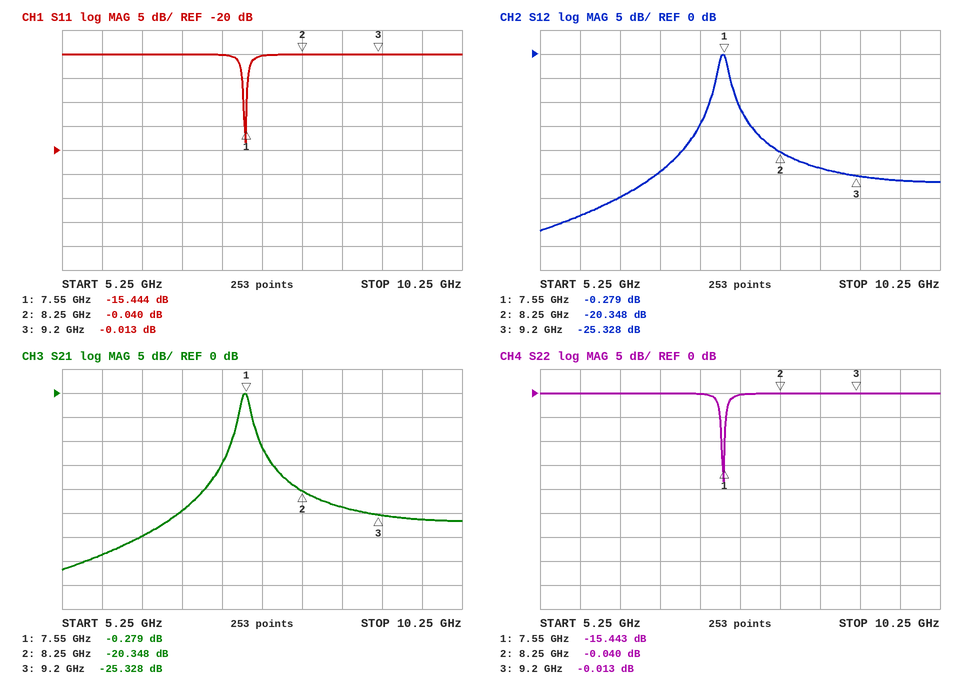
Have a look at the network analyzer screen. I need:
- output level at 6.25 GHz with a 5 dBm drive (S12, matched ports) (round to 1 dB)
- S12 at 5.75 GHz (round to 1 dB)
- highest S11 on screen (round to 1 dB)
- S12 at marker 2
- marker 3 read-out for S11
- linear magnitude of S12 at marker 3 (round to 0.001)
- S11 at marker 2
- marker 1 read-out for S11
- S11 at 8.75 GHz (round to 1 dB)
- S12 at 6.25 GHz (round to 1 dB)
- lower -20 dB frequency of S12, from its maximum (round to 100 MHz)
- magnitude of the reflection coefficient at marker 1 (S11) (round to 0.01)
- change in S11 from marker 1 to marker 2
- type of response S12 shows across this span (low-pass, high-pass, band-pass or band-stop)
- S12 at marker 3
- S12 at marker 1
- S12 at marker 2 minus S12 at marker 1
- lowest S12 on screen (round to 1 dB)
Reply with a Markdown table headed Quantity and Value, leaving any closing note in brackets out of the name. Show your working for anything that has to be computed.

| Quantity | Value |
|---|---|
| output level at 6.25 GHz with a 5 dBm drive (S12, matched ports) | 5 dBm + (-30 dB) = -25 dBm |
| S12 at 5.75 GHz | -34 dB |
| highest S11 on screen | 0 dB |
| S12 at marker 2 | -20.348 dB |
| marker 3 read-out for S11 | -0.013 dB |
| linear magnitude of S12 at marker 3 | 10^(-25.328/20) ≈ 0.054 |
| S11 at marker 2 | -0.040 dB |
| marker 1 read-out for S11 | -15.444 dB |
| S11 at 8.75 GHz | 0 dB |
| S12 at 6.25 GHz | -30 dB |
| lower -20 dB frequency of S12, from its maximum | 7.0 GHz |
| magnitude of the reflection coefficient at marker 1 (S11) | 10^(-15.444/20) ≈ 0.17 |
| change in S11 from marker 1 to marker 2 | -0.04 − (-15.444) = 15.404 dB |
| type of response S12 shows across this span | band-pass |
| S12 at marker 3 | -25.328 dB |
| S12 at marker 1 | -0.279 dB |
| S12 at marker 2 minus S12 at marker 1 | -20.348 − (-0.279) = -20.069 dB |
| lowest S12 on screen | -37 dB |
